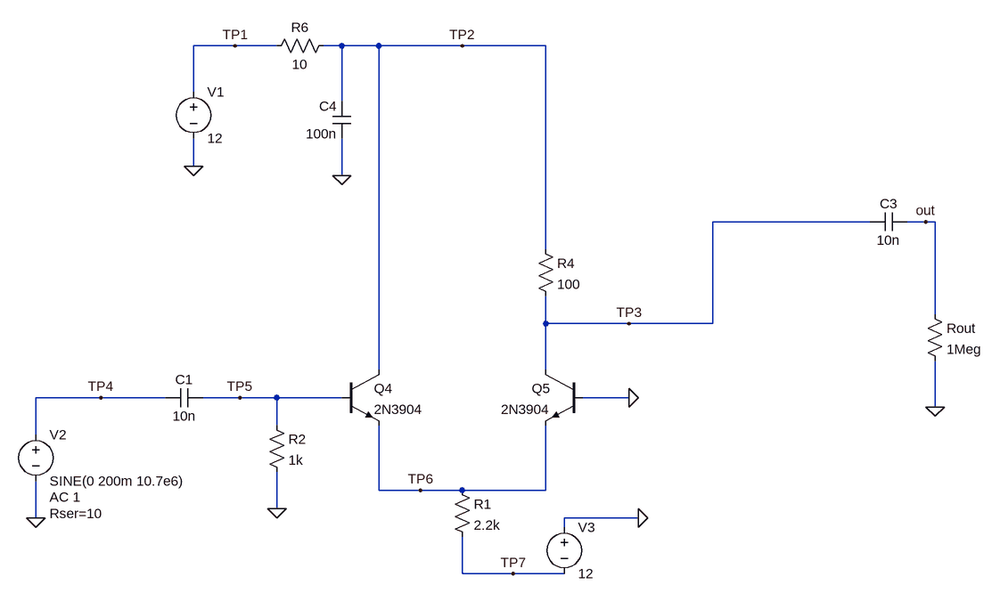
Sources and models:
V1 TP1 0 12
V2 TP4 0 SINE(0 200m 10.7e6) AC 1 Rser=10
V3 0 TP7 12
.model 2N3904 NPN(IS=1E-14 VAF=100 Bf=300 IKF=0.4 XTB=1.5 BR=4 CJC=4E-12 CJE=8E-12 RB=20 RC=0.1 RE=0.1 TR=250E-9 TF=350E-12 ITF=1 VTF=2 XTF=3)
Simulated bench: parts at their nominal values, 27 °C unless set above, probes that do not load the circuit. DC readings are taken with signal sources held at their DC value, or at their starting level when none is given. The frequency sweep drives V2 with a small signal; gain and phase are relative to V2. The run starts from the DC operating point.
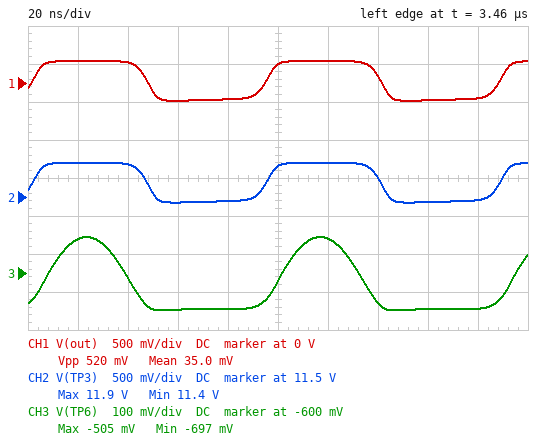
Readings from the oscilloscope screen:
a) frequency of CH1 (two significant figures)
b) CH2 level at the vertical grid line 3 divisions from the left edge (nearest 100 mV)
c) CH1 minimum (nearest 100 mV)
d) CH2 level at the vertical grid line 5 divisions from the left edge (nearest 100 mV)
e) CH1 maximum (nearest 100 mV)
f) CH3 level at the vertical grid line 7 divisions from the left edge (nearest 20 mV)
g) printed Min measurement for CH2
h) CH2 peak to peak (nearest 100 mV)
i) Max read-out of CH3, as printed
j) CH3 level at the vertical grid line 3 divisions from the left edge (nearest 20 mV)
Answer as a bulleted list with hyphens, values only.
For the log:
- 11 MHz
- 11.4 V
- -200 mV
- 11.9 V
- 300 mV
- -680 mV
- 11.4 V
- 500 mV
- -505 mV
- -700 mV
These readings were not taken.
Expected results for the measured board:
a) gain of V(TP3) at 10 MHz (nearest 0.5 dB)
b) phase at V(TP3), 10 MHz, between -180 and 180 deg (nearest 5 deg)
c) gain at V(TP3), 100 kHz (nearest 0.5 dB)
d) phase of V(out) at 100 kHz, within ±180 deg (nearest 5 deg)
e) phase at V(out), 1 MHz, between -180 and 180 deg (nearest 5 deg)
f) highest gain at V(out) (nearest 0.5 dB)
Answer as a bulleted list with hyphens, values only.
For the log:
- 13.5 dB
- -5 deg
- 13.5 dB
- 10 deg
- 0 deg
- 13.5 dB
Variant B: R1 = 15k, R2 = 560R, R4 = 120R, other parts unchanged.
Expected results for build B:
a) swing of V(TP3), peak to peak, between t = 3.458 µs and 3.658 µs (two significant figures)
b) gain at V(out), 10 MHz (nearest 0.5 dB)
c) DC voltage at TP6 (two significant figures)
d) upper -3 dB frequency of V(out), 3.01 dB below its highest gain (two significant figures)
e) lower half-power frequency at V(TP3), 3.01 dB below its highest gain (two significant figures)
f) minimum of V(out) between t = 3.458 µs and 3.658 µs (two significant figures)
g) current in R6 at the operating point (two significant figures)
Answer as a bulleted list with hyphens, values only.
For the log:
- 100 mV
- -1.5 dB
- -630 mV
- 230 MHz
- 28 kHz
- -58 mV
- 760 µA
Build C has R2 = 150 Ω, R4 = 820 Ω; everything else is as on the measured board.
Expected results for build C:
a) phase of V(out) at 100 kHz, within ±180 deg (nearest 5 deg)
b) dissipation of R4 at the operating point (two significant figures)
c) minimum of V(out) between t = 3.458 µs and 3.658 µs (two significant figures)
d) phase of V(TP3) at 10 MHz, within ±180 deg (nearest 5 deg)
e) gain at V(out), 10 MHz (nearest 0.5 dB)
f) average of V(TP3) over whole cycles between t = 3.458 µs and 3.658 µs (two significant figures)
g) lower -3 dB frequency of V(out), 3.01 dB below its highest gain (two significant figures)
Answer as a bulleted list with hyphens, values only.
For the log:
- 45 deg
- 5.5 mW
- -2.1 V
- -15 deg
- 31.0 dB
- 9.8 V
- 100 kHz
